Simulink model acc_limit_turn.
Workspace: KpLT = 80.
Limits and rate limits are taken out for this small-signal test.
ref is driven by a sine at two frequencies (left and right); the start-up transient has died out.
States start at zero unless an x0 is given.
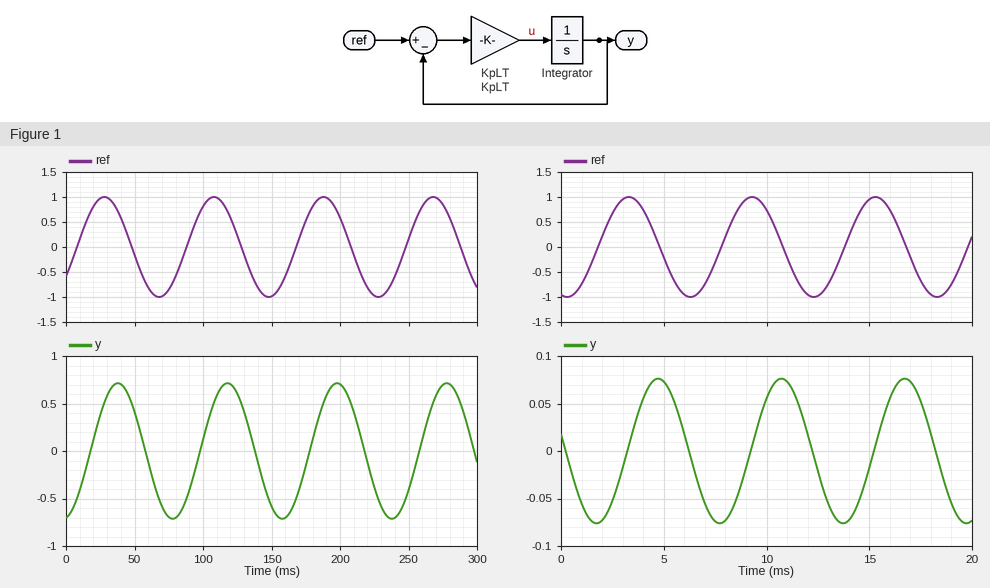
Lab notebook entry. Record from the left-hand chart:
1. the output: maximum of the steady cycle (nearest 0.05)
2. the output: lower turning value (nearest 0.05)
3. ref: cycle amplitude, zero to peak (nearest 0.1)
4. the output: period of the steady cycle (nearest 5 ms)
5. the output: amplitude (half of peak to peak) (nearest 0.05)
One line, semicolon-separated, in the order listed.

0.70; -0.70; 1.0; 80 ms; 0.70
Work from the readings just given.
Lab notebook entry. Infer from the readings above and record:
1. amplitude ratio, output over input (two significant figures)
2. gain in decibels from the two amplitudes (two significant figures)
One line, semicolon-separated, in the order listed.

0.70; -3.1 dB
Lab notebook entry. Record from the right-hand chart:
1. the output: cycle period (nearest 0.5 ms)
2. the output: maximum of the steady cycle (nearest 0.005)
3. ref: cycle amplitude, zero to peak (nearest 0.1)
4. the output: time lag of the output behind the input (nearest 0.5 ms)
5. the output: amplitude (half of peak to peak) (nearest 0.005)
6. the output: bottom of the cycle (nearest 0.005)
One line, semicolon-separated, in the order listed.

6.0 ms; 0.075; 1.0; 1.5 ms; 0.075; -0.075
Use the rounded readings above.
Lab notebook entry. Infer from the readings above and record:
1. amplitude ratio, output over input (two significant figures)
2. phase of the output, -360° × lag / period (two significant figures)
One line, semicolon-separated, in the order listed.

0.075; -90°
